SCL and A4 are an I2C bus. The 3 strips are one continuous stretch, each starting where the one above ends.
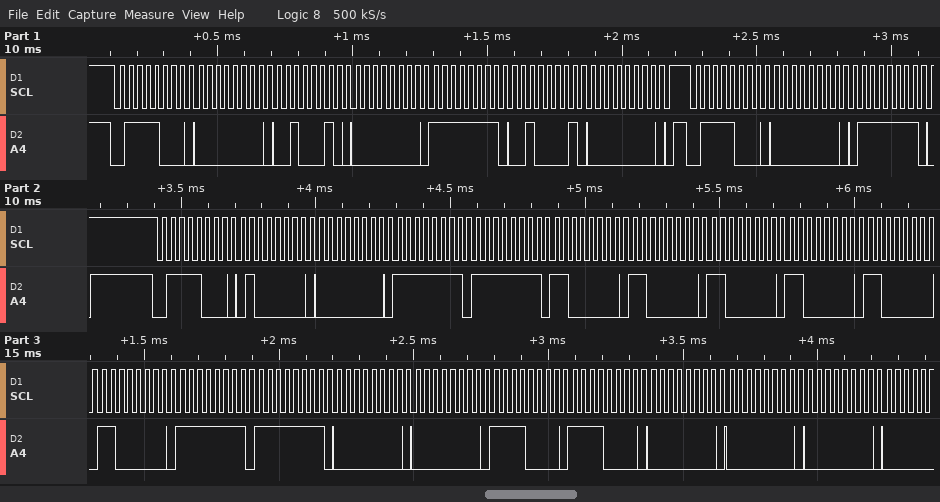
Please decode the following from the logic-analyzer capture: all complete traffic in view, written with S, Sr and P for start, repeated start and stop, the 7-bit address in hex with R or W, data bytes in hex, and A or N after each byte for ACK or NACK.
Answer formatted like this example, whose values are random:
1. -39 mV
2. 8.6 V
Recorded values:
1. S 3CW A 00 A 22 A 00 A FF A 21 A 00 A P S 3CW A 00 A 7F A P S 3CW A 40 A 00 A FF A FF A C0 A C0 A C0 A C0 A C0 A C0 A FF A FF A 00 A 00 A F0 A F0 A 00 A 00 A 00 A
